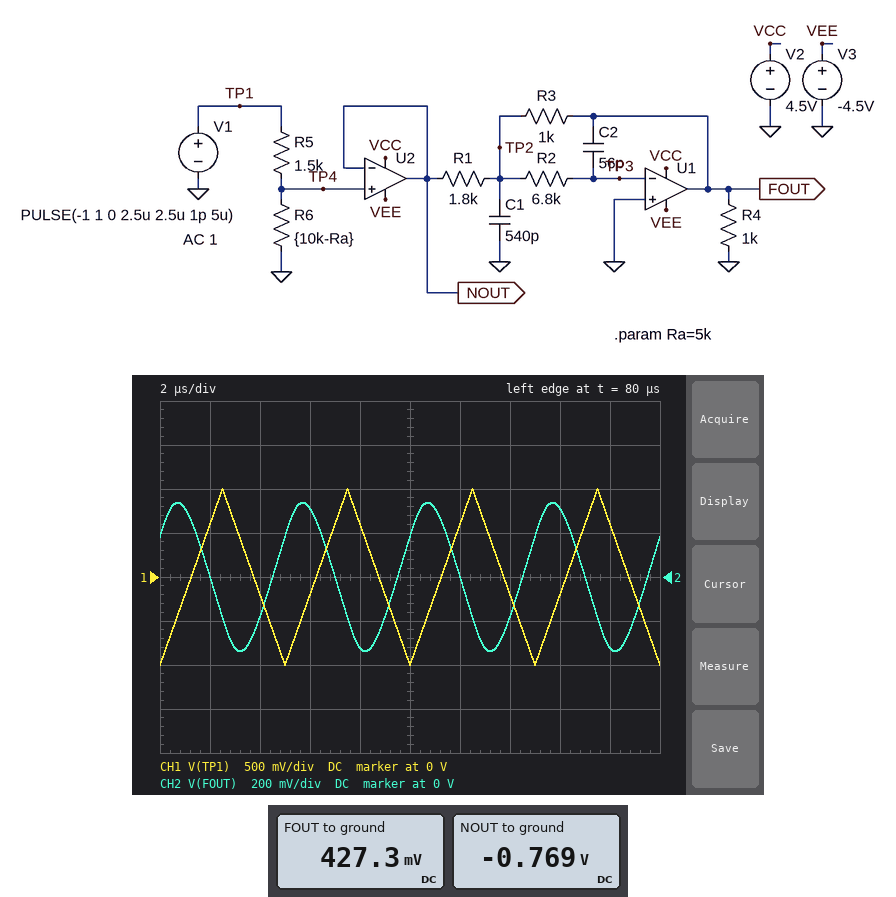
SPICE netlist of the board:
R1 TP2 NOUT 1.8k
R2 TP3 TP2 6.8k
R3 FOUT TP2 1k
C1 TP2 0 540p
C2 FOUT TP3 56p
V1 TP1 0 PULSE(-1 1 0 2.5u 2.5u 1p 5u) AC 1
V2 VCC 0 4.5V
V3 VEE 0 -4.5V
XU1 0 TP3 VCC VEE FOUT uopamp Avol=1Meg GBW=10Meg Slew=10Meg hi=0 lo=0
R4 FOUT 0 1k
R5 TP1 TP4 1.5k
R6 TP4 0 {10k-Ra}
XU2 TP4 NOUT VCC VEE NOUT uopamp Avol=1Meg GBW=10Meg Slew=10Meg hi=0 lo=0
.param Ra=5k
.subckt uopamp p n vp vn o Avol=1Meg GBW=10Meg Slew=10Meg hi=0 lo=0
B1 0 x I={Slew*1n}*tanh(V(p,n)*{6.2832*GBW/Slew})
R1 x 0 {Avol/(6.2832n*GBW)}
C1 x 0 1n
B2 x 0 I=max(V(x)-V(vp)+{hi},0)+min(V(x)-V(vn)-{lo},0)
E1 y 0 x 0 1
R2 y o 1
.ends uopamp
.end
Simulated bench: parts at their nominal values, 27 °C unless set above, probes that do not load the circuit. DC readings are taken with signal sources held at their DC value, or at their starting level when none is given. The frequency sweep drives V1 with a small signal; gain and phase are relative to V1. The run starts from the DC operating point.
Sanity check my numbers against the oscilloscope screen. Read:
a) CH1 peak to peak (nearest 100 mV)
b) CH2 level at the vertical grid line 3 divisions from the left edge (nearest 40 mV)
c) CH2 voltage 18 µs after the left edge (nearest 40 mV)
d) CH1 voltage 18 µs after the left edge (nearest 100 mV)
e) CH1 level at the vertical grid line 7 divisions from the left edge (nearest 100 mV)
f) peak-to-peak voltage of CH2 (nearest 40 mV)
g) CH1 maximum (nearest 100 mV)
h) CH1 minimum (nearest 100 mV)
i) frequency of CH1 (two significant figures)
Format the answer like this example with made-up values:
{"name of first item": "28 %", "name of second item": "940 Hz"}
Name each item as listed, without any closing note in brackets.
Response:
{"CH1 peak to peak": "2.0 V", "CH2 level at the vertical grid line 3 divisions from the left edge": "320 mV", "CH2 voltage 18 µs after the left edge": "-320 mV", "CH1 voltage 18 µs after the left edge": "600 mV", "CH1 level at the vertical grid line 7 divisions from the left edge": "-200 mV", "peak-to-peak voltage of CH2": "680 mV", "CH1 maximum": "1.0 V", "CH1 minimum": "-1.0 V", "frequency of CH1": "200 kHz"}
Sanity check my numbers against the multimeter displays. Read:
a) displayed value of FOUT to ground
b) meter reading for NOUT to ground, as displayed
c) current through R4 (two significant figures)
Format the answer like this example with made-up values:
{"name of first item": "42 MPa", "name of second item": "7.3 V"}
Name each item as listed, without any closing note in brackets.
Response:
{"displayed value of FOUT to ground": "427.3 mV", "meter reading for NOUT to ground, as displayed": "-0.769 V", "current through R4": "430 µA"}
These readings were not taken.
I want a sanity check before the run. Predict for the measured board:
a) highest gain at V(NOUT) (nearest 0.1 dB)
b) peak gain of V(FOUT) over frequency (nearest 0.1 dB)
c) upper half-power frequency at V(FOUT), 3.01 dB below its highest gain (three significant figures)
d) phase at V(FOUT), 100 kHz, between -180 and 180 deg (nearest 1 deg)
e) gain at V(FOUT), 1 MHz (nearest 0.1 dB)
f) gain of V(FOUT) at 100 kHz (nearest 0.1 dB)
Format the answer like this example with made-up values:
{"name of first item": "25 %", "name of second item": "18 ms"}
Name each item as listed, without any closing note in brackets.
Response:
{"highest gain at V(NOUT)": "-2.3 dB", "peak gain of V(FOUT) over frequency": "-7.4 dB", "upper half-power frequency at V(FOUT), 3.01 dB below its highest gain": "342 kHz", "phase at V(FOUT), 100 kHz, between -180 and 180 deg": "155 deg", "gain at V(FOUT), 1 MHz": "-26.1 dB", "gain of V(FOUT) at 100 kHz": "-7.4 dB"}
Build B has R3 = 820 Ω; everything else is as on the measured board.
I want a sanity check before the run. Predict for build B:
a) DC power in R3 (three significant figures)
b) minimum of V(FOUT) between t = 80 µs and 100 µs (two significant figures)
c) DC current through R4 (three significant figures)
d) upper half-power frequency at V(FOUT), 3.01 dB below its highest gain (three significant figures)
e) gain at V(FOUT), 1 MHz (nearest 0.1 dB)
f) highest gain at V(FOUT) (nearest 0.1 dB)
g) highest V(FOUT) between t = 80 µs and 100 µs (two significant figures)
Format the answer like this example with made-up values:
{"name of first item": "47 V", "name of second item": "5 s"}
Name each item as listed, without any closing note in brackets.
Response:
{"DC power in R3": "150 µW", "minimum of V(FOUT) between t = 80 µs and 100 µs": "-280 mV", "DC current through R4": "350 µA", "upper half-power frequency at V(FOUT), 3.01 dB below its highest gain": "369 kHz", "gain at V(FOUT), 1 MHz": "-26.2 dB", "highest gain at V(FOUT)": "-9.1 dB", "highest V(FOUT) between t = 80 µs and 100 µs": "280 mV"}
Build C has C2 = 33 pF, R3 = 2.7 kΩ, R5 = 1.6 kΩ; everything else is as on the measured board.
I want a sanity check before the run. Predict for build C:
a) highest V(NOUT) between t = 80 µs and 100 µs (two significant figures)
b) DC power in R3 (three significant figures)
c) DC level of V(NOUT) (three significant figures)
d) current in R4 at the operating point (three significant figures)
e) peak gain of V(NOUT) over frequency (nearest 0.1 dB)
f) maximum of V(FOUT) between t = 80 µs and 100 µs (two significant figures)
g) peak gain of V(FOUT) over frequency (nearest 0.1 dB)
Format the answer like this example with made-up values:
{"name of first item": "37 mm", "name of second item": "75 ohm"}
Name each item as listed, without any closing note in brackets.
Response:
{"highest V(NOUT) between t = 80 µs and 100 µs": "750 mV", "DC power in R3": "478 µW", "DC level of V(NOUT)": "-758 mV", "current in R4 at the operating point": "1.14 mA", "peak gain of V(NOUT) over frequency": "-2.4 dB", "maximum of V(FOUT) between t = 80 µs and 100 µs": "980 mV", "peak gain of V(FOUT) over frequency": "1.7 dB"}
